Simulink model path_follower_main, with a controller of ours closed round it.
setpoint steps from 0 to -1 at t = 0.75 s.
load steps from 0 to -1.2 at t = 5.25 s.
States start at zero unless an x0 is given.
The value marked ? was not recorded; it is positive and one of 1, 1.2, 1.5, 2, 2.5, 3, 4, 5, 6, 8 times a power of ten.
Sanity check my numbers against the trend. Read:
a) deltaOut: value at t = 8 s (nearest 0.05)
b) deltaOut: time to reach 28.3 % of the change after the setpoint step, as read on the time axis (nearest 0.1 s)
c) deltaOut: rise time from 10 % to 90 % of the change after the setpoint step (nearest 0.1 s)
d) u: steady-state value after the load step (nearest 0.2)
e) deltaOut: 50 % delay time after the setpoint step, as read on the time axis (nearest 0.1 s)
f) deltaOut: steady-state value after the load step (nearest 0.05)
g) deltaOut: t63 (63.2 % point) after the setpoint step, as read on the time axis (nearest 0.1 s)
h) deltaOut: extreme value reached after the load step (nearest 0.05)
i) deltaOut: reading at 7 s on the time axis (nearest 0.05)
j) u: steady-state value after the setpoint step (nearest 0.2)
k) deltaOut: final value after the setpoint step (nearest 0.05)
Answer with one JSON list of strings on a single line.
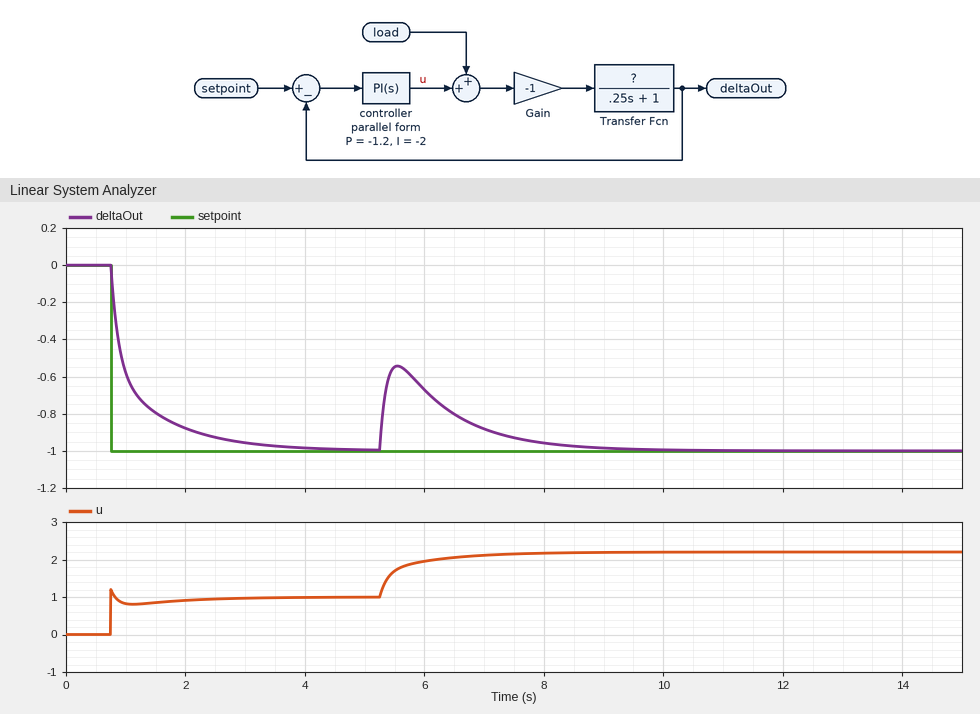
["-0.95", "0.8 s", "1.4 s", "2.2", "0.9 s", "-1.00", "1.1 s", "-0.55", "-0.90", "1.0", "-1.00"]
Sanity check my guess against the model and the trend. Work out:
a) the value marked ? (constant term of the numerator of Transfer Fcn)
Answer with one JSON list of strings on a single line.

["1"]
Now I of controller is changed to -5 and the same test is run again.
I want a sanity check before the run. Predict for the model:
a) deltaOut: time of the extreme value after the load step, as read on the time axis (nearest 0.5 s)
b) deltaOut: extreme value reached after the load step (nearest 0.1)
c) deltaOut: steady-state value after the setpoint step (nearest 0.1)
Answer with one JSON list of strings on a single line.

["5.5 s", "-0.6", "-1.0"]
